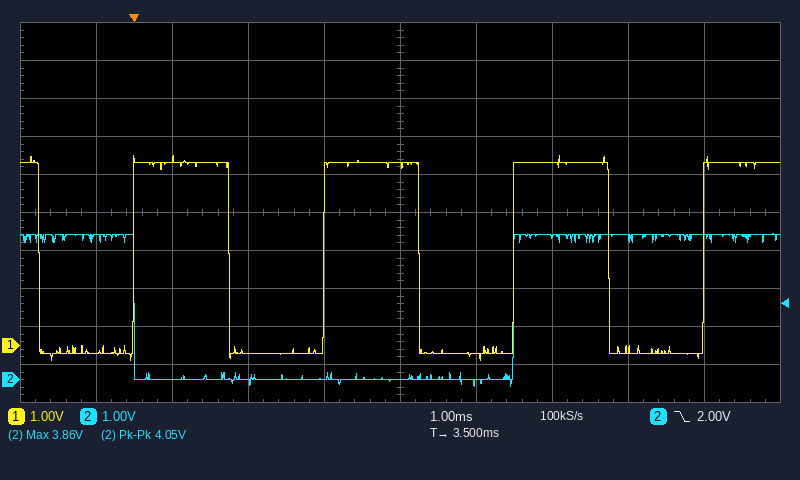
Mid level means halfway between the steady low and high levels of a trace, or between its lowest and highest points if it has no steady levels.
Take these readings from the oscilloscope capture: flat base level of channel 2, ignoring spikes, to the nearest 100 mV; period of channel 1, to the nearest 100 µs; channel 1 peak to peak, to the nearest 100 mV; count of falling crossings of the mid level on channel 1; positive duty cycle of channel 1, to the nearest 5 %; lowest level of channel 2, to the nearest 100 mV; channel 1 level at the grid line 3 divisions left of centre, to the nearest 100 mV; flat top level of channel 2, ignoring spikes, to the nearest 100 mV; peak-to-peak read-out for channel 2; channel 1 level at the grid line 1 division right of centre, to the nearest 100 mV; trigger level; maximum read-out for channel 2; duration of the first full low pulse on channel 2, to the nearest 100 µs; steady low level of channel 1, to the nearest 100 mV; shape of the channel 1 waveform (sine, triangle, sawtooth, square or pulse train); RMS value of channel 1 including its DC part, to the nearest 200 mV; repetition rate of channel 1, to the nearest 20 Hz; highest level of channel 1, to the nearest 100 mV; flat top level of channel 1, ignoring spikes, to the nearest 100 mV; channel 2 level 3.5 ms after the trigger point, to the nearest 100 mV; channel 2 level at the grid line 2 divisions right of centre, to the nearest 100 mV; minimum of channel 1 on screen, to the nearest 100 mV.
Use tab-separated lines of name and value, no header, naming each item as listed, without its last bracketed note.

flat base level of channel 2, ignoring spikes, to the nearest 100 mV	0.0 V
period of channel 1, to the nearest 100 µs	2.5 ms
channel 1 peak to peak, to the nearest 100 mV	5.4 V
count of falling crossings of the mid level on channel 1	4
positive duty cycle of channel 1, to the nearest 5 %	50 %
lowest level of channel 2, to the nearest 100 mV	-200 mV
channel 1 level at the grid line 3 divisions left of centre, to the nearest 100 mV	4.9 V
flat top level of channel 2, ignoring spikes, to the nearest 100 mV	3.8 V
peak-to-peak read-out for channel 2	4.05 V
channel 1 level at the grid line 1 division right of centre, to the nearest 100 mV	-300 mV
trigger level	2.00 V
maximum read-out for channel 2	3.86 V
duration of the first full low pulse on channel 2, to the nearest 100 µs	5.0 ms
steady low level of channel 1, to the nearest 100 mV	-200 mV
shape of the channel 1 waveform	square
RMS value of channel 1 including its DC part, to the nearest 200 mV	3.4 V
repetition rate of channel 1, to the nearest 20 Hz	400 Hz
highest level of channel 1, to the nearest 100 mV	5.0 V
flat top level of channel 1, ignoring spikes, to the nearest 100 mV	4.8 V
channel 2 level 3.5 ms after the trigger point, to the nearest 100 mV	0.0 V
channel 2 level at the grid line 2 divisions right of centre, to the nearest 100 mV	3.8 V
minimum of channel 1 on screen, to the nearest 100 mV	-400 mV
